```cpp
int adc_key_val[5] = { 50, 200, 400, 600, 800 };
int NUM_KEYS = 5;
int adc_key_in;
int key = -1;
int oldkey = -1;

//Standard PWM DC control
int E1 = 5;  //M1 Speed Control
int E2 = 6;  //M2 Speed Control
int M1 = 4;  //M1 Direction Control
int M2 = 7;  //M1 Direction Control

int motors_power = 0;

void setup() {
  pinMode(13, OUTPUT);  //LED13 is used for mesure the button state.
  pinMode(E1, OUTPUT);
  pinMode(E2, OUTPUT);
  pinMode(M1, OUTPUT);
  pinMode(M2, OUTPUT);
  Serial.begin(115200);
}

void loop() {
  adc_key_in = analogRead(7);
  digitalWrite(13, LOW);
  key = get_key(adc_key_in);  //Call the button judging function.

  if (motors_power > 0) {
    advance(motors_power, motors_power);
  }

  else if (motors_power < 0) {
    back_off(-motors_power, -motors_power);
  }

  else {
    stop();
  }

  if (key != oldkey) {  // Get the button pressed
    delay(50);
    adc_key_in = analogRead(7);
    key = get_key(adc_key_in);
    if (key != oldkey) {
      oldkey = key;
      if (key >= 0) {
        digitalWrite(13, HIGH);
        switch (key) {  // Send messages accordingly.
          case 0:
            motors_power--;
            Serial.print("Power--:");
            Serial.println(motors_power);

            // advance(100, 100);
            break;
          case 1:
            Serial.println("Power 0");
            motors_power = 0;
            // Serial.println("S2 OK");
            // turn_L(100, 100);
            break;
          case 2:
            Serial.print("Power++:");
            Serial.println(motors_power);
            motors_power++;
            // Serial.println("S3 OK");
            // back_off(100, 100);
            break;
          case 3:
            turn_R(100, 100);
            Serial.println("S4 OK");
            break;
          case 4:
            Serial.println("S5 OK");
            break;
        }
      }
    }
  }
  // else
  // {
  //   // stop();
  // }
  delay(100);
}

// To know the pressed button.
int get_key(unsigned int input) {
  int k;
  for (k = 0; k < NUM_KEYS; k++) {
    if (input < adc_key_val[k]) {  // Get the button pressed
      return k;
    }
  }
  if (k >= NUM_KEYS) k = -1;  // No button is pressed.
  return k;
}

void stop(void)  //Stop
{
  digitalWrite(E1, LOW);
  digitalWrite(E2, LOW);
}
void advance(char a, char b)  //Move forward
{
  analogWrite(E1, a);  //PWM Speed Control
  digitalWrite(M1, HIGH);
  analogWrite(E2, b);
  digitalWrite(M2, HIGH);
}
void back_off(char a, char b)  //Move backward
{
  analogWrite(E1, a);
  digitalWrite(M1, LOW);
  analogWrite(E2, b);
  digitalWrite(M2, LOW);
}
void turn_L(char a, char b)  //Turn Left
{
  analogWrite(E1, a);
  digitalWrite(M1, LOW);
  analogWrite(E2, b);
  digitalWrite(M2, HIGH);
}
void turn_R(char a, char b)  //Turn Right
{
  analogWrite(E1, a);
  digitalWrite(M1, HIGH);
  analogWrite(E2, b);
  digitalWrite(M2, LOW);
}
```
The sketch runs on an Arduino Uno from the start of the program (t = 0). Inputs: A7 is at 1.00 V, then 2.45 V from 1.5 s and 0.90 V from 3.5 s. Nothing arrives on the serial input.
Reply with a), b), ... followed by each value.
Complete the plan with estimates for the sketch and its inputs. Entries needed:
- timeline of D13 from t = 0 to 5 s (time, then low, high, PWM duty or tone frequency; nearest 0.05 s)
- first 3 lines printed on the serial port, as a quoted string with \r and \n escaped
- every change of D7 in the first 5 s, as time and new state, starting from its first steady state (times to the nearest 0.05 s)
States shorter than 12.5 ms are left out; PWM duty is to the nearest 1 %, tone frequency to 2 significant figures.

a) 0 s low; 0.05 s high; 0.15 s low; 1.6 s high; 1.7 s low; 3.55 s high; 3.65 s low
b) "Power++:0\r\nS4 OK\r\nPower 0\r\n"
c) 0 s low; 0.15 s high; 1.6 s low; 1.7 s high
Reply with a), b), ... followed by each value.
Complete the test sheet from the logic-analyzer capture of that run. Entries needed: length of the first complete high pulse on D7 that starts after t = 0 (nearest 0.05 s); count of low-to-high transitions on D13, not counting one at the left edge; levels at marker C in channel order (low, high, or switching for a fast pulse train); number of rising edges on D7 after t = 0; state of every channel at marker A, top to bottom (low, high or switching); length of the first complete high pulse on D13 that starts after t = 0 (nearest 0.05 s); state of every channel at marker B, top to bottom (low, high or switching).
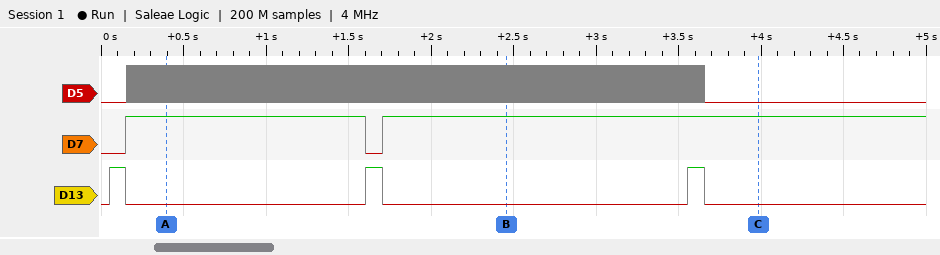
a) 1.45 s
b) 3
c) D5 low, D7 high, D13 low
d) 2
e) D5 switching, D7 high, D13 low
f) 0.10 s
g) D5 switching, D7 high, D13 low
